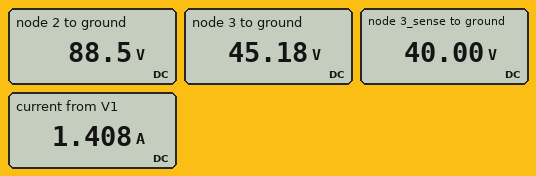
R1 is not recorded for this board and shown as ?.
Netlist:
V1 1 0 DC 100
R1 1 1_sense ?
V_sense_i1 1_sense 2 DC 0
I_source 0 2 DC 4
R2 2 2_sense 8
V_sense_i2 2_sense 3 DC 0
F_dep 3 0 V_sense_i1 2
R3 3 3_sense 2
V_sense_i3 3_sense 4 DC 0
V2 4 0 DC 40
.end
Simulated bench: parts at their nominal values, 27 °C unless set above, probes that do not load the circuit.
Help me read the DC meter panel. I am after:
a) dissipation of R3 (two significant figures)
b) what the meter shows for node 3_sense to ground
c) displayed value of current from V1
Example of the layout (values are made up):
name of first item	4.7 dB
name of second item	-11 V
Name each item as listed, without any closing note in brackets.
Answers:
dissipation of R3	13 W
what the meter shows for node 3_sense to ground	40.00 V
displayed value of current from V1	1.408 A
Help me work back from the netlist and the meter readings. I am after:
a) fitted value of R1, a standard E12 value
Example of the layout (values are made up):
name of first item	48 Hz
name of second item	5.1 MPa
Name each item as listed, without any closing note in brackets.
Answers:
fitted value of R1, a standard E12 value	8.2 Ω
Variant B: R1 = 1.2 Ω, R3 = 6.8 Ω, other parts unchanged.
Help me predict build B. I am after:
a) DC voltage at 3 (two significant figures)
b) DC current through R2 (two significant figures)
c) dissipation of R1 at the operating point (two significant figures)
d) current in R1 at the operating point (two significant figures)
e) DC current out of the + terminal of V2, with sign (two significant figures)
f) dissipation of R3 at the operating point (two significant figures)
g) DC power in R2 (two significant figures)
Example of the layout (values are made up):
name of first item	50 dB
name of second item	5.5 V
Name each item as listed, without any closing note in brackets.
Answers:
DC voltage at 3	65 V
DC current through R2	4.3 A
dissipation of R1 at the operating point	130 mW
current in R1 at the operating point	330 mA
DC current out of the + terminal of V2, with sign	-3.7 A
dissipation of R3 at the operating point	91 W
DC power in R2	150 W
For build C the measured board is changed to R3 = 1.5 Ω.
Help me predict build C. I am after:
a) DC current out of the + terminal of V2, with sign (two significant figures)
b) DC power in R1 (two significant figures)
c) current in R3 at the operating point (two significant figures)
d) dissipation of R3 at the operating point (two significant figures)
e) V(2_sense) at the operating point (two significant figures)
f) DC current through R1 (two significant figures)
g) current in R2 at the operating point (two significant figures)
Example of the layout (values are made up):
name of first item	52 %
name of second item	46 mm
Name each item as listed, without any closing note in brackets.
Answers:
DC current out of the + terminal of V2, with sign	-2.5 A
DC power in R1	18 W
current in R3 at the operating point	2.5 A
dissipation of R3 at the operating point	9.4 W
V(2_sense) at the operating point	44 V
DC current through R1	1.5 A
current in R2 at the operating point	5.5 A
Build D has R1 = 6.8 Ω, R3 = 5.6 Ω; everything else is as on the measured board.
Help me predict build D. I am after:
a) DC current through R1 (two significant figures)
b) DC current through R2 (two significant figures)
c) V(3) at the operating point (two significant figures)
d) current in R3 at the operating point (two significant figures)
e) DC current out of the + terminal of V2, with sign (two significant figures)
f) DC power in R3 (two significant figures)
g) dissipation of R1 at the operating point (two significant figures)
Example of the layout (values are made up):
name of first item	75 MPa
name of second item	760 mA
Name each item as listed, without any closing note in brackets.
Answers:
DC current through R1	610 mA
DC current through R2	4.6 A
V(3) at the operating point	59 V
current in R3 at the operating point	3.4 A
DC current out of the + terminal of V2, with sign	-3.4 A
DC power in R3	64 W
dissipation of R1 at the operating point	2.5 W
